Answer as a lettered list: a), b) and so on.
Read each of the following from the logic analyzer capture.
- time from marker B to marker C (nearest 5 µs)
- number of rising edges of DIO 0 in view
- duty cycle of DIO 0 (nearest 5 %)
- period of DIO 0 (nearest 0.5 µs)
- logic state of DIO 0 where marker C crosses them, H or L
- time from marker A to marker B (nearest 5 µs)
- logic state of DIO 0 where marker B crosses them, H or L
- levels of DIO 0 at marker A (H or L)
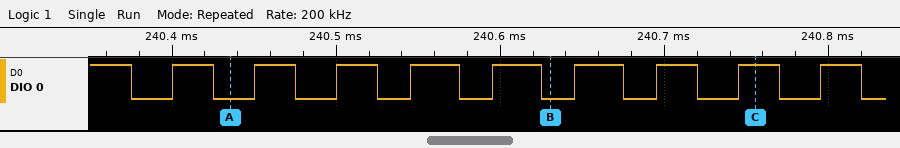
a) 125 µs
b) 9
c) 55 %
d) 49.5 µs
e) DIO 0=H
f) 195 µs
g) DIO 0=L
h) DIO 0=L
